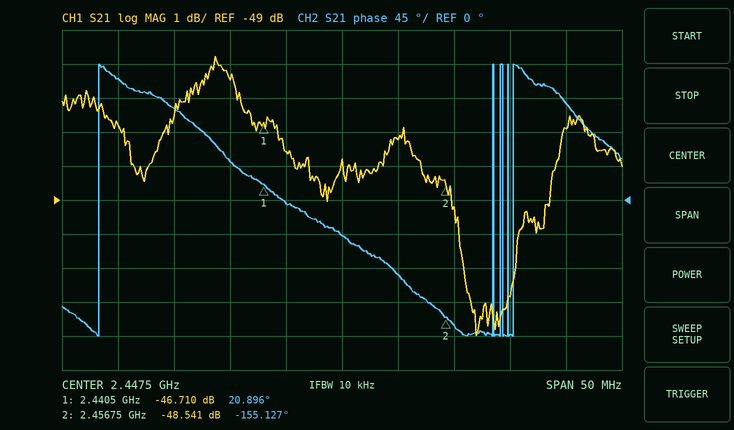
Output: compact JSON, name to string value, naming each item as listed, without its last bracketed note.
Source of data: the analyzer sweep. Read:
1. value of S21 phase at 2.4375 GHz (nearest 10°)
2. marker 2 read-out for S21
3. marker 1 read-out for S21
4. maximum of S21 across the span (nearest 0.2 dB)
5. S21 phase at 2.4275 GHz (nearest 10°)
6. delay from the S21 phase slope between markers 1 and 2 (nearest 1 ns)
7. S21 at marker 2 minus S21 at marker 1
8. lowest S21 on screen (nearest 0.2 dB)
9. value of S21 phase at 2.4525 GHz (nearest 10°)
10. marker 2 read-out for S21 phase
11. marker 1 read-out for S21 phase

{"value of S21 phase at 2.4375 GHz": "50°", "marker 2 read-out for S21": "-48.541 dB", "marker 1 read-out for S21": "-46.710 dB", "maximum of S21 across the span": "-44.8 dB", "S21 phase at 2.4275 GHz": "160°", "delay from the S21 phase slope between markers 1 and 2": "30 ns", "S21 at marker 2 minus S21 at marker 1": "-1.831 dB", "lowest S21 on screen": "-53.0 dB", "value of S21 phase at 2.4525 GHz": "-100°", "marker 2 read-out for S21 phase": "-155.127°", "marker 1 read-out for S21 phase": "20.896°"}
